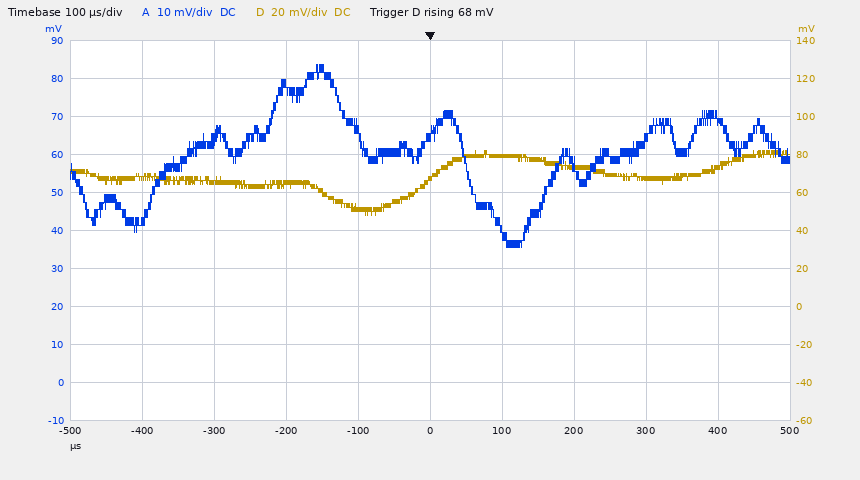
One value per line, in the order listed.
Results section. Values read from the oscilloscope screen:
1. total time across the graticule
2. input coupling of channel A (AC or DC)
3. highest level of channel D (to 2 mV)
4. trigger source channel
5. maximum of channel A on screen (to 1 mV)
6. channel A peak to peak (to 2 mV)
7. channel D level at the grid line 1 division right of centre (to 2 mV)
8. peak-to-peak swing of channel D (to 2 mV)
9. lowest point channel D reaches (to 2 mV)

1 ms
DC
82 mV
channel D
84 mV
48 mV
80 mV
34 mV
48 mV
